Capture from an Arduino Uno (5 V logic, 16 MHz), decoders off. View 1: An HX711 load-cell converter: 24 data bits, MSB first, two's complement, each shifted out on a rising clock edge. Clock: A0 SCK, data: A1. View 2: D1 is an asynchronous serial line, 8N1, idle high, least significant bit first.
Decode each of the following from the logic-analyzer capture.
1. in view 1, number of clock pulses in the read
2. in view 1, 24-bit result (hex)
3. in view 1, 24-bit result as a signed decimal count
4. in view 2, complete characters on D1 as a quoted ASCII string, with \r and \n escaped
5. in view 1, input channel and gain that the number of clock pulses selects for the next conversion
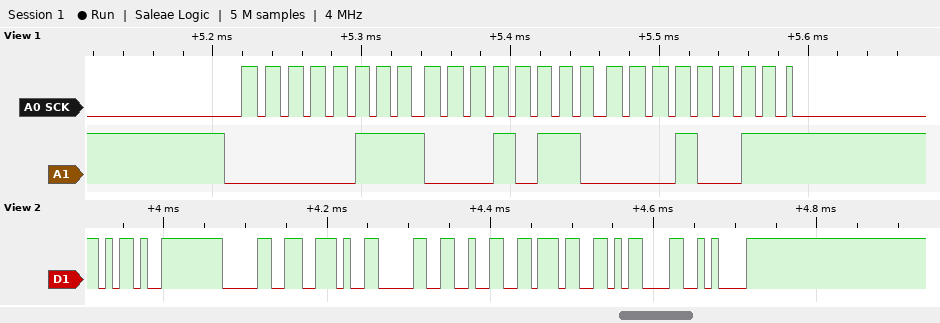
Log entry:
25
0x071613
464403
"-0.027\r\n"
channel A, gain 128
